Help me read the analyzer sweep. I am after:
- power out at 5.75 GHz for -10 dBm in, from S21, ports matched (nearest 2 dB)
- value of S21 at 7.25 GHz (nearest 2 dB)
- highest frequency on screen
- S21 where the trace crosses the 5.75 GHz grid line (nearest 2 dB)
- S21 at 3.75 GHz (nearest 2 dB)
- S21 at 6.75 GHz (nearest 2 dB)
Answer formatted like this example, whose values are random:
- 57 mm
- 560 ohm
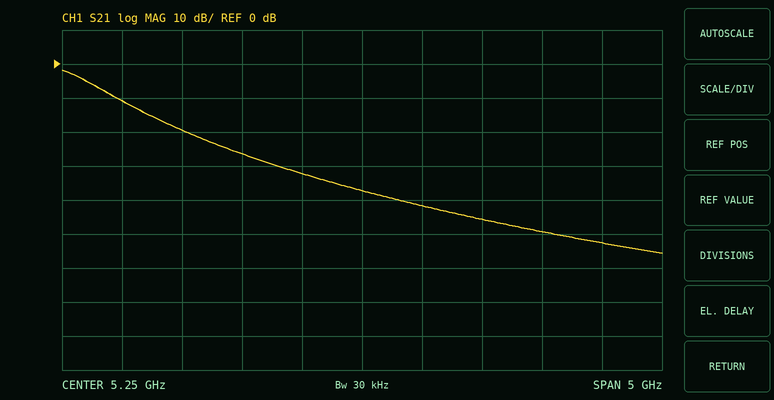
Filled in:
- -52 dBm
- -52 dB
- 7.75 GHz
- -42 dB
- -20 dB
- -50 dB
